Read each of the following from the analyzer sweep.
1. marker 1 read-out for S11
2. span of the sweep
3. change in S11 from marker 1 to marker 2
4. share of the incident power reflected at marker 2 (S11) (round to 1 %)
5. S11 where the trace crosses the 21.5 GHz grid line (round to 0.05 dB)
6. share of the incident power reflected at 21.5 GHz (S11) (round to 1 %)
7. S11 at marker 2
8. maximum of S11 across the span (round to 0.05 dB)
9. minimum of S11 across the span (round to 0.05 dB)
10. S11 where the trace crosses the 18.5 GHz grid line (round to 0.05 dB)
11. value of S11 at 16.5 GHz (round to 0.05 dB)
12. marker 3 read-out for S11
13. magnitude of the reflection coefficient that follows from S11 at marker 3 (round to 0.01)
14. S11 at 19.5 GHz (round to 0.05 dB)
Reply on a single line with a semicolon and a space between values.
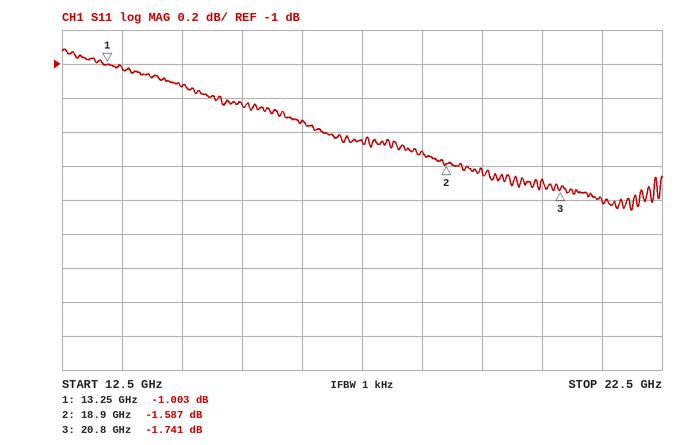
-1.003 dB; 10 GHz; -0.584 dB; 69 %; -1.80 dB; 66 %; -1.587 dB; -0.90 dB; -1.85 dB; -1.50 dB; -1.35 dB; -1.741 dB; 0.82; -1.65 dB
